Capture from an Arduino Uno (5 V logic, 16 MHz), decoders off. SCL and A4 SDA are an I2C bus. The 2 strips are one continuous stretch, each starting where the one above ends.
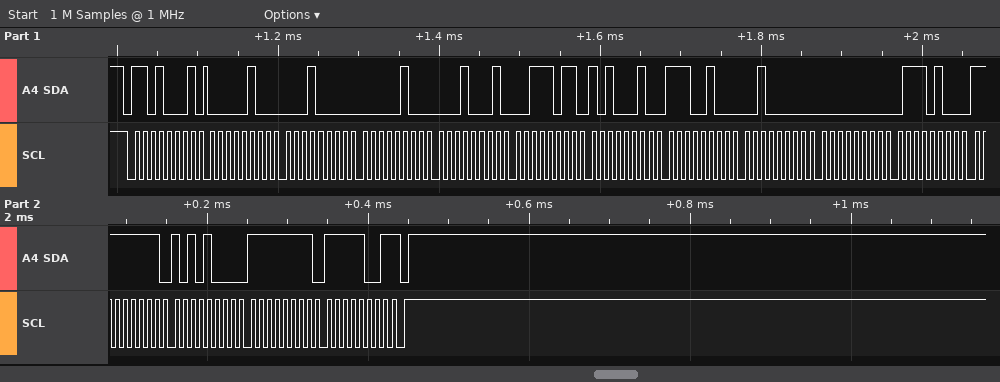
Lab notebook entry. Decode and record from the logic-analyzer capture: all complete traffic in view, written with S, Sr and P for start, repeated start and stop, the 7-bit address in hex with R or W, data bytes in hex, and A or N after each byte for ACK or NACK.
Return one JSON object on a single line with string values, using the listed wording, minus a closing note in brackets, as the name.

{"all complete traffic in view, written with S, Sr and P for start, repeated start and stop, the 7-bit address in hex with R or W, data bytes in hex, and A or N after each byte for ACK or NACK": "S 68R A 04 A 10 A 04 A 11 A 3B A A2 A E4 A 20 A 00 A 74 A FF A A8 A FF A F9 N P"}
